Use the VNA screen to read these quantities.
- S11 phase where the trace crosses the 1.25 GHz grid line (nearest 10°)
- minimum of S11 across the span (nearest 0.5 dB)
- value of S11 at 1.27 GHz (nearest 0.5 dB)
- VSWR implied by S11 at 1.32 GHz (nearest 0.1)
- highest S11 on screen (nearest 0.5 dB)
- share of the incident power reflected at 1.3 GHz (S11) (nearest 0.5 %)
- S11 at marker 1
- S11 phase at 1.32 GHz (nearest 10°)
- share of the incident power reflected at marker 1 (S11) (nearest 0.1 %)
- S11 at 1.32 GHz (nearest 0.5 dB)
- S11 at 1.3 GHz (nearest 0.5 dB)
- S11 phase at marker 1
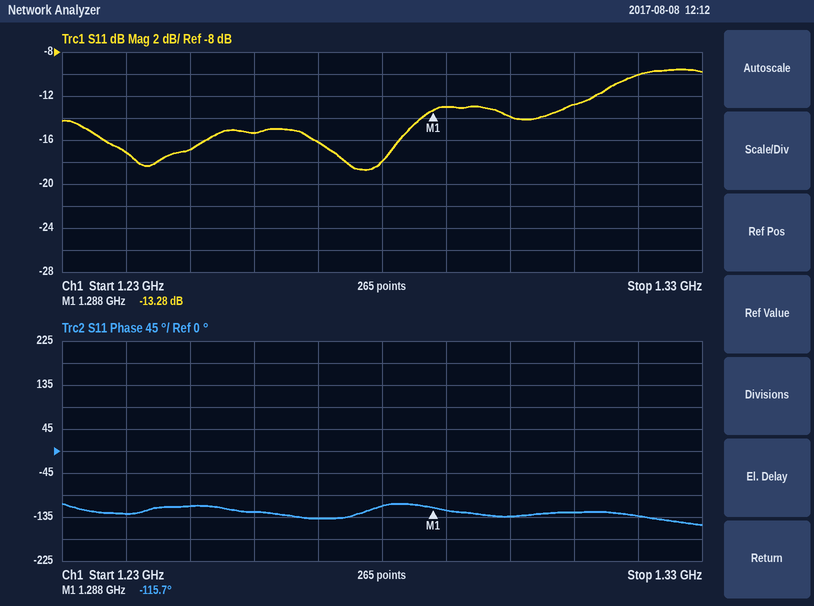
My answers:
-110°
-18.5 dB
-16.0 dB
1.9
-9.5 dB
4.0 %
-13.28 dB
-130°
4.7 %
-10.0 dB
-14.0 dB
-115.7°
